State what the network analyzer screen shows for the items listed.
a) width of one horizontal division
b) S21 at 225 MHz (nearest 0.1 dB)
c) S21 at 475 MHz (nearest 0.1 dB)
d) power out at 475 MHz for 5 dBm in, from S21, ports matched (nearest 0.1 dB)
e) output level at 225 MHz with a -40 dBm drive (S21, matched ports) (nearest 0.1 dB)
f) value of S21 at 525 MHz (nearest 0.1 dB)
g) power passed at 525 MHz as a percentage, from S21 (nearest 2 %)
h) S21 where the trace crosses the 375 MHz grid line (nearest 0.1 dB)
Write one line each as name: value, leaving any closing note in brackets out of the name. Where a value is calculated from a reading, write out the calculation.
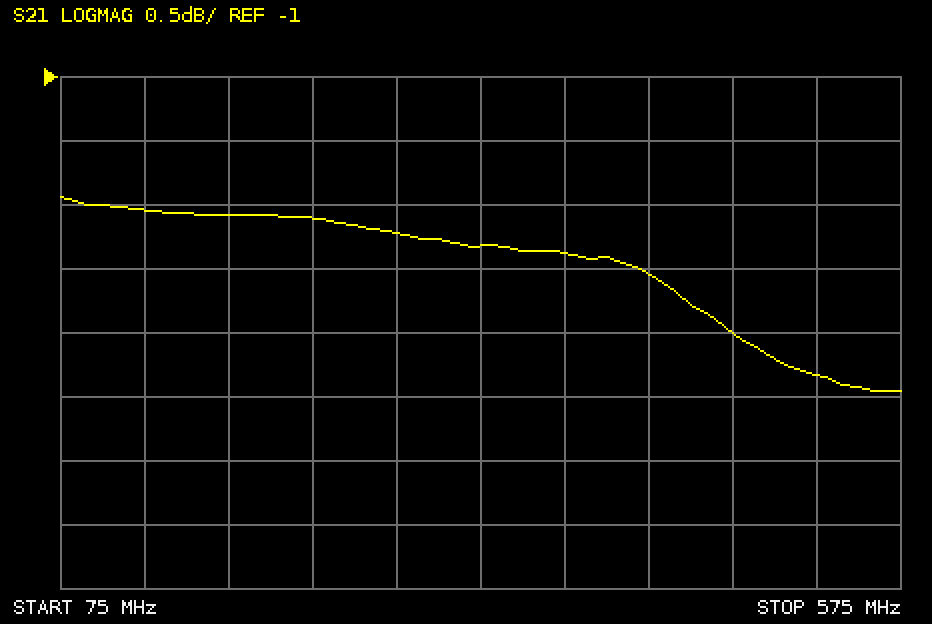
width of one horizontal division: 50 MHz
S21 at 225 MHz: -2.1 dB
S21 at 475 MHz: -3.0 dB
power out at 475 MHz for 5 dBm in, from S21, ports matched: 5 dBm + (-3.0 dB) = 2.0 dBm
output level at 225 MHz with a -40 dBm drive (S21, matched ports): -40 dBm + (-2.1 dB) = -42.1 dBm
value of S21 at 525 MHz: -3.3 dB
power passed at 525 MHz as a percentage, from S21: 10^(-3.3/10) ≈ 46.8 %, so 46 % to the nearest 2 %
S21 where the trace crosses the 375 MHz grid line: -2.4 dB
